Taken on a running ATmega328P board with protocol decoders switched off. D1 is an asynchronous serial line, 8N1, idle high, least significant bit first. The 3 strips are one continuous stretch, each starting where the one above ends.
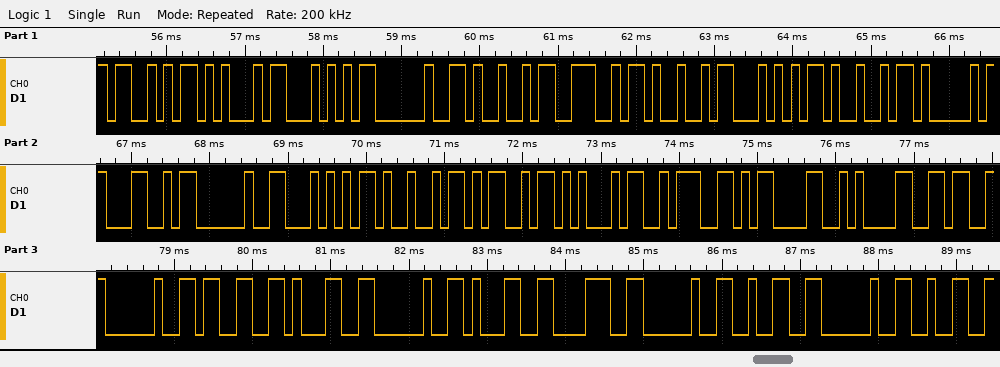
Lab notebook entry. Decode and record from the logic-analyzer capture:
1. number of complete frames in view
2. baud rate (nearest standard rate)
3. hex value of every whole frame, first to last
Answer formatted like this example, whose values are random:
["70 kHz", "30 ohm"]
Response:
["30", "9600 baud", "53 45 54 20 49 4E 49 54 49 41 4C 20 54 49 4D 45 3A 0D 0A 36 20 33 31 20 31 38 20 32 20 32"]
